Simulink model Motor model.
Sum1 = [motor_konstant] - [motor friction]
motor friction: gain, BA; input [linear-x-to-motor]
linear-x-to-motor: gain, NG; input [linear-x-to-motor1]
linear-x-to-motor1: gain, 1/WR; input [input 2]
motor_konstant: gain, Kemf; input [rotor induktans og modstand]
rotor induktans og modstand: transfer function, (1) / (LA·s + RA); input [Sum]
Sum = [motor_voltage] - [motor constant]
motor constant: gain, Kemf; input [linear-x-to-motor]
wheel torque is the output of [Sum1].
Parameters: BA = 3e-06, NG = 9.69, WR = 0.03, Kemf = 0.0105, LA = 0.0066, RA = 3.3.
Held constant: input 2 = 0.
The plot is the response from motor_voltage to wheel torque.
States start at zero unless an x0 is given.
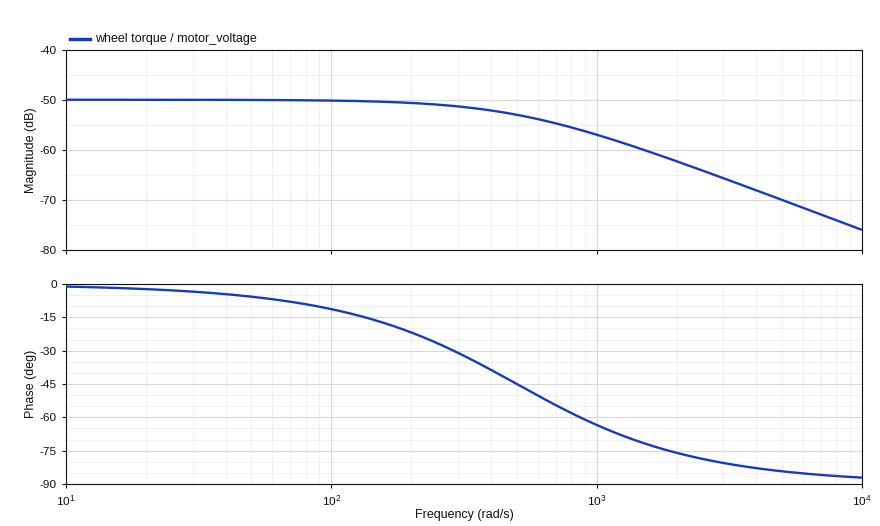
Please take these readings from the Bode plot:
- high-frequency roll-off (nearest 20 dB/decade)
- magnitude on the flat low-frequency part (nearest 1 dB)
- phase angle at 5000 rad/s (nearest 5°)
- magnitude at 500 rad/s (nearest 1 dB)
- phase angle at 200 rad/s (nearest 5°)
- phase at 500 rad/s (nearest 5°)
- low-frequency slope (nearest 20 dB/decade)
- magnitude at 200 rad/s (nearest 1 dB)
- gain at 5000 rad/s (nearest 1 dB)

-20 dB/decade
-50 dB
-85°
-53 dB
-20°
-45°
0 dB/decade
-51 dB
-70 dB
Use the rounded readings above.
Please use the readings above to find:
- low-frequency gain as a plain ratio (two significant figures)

0.0032
